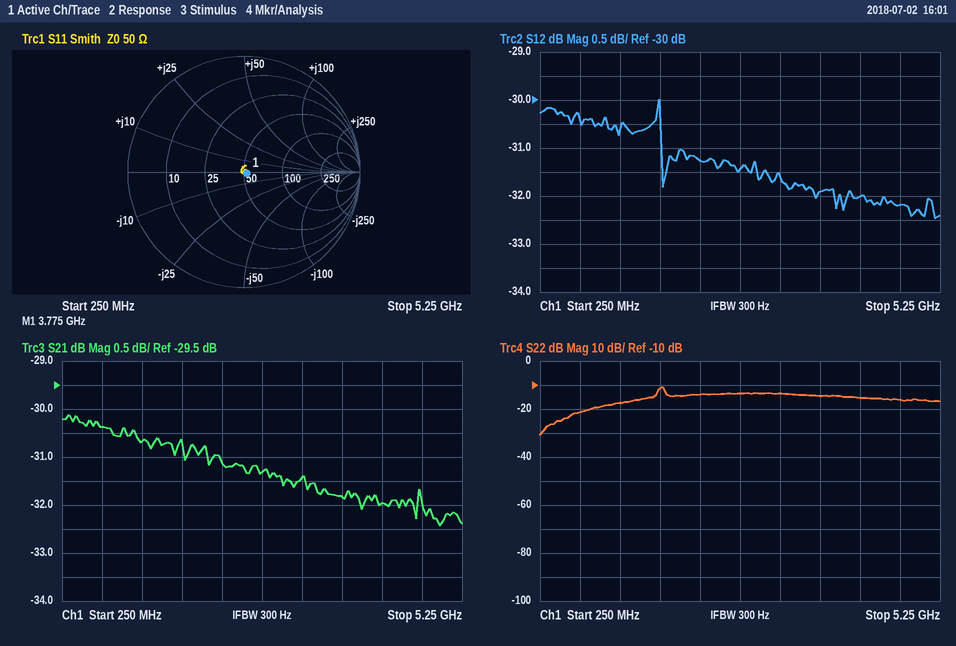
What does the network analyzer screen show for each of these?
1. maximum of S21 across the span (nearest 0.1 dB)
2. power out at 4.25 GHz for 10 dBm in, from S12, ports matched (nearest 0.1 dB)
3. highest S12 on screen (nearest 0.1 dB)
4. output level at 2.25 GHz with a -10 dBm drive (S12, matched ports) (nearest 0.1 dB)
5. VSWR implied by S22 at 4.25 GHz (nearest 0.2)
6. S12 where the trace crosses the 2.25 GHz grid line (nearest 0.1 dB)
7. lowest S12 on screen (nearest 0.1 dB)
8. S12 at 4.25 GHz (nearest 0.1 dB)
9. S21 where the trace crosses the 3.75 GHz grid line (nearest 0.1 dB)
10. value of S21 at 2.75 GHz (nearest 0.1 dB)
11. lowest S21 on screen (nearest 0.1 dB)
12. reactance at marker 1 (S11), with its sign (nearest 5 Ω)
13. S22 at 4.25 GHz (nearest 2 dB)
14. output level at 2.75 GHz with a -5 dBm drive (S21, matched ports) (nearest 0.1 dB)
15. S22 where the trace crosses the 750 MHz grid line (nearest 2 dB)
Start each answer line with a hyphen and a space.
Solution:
- -30.1 dB
- -22.0 dBm
- -30.0 dB
- -41.3 dBm
- 1.4
- -31.3 dB
- -32.5 dB
- -32.0 dB
- -31.8 dB
- -31.3 dB
- -32.4 dB
- 0 Ω
- -16 dB
- -36.3 dBm
- -22 dB
